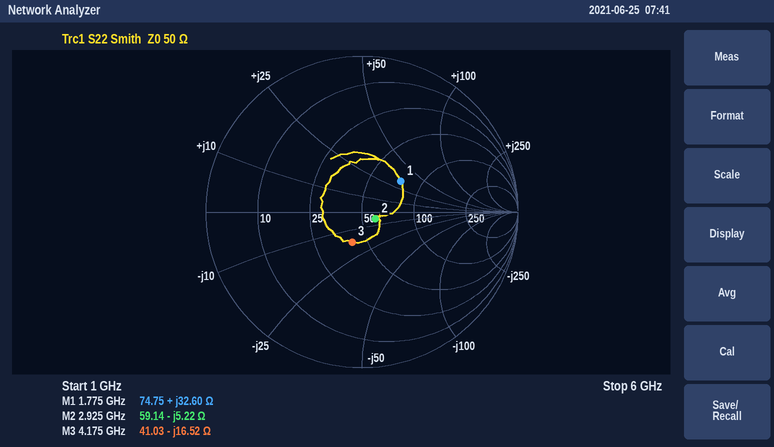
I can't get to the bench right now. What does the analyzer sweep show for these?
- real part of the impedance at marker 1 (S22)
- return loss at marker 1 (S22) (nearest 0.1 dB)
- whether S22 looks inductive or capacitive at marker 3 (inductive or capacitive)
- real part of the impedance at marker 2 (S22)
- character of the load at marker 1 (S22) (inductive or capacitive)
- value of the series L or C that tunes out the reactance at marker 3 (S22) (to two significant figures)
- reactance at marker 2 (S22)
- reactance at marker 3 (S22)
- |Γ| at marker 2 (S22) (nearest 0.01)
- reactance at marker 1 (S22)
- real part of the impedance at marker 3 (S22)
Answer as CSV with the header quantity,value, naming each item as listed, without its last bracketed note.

quantity,value
real part of the impedance at marker 1,74.75 Ω
return loss at marker 1 (S22),10.0 dB
whether S22 looks inductive or capacitive at marker 3,capacitive
real part of the impedance at marker 2,59.14 Ω
character of the load at marker 1 (S22),inductive
value of the series L or C that tunes out the reactance at marker 3 (S22),630 pH
reactance at marker 2,-5.22 Ω
reactance at marker 3,-16.52 Ω
|Γ| at marker 2 (S22),0.10
reactance at marker 1,+32.60 Ω
real part of the impedance at marker 3,41.03 Ω
